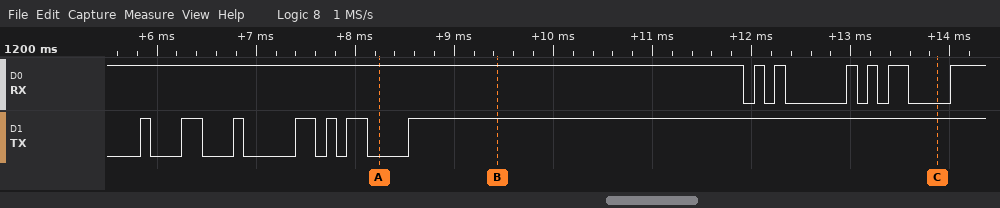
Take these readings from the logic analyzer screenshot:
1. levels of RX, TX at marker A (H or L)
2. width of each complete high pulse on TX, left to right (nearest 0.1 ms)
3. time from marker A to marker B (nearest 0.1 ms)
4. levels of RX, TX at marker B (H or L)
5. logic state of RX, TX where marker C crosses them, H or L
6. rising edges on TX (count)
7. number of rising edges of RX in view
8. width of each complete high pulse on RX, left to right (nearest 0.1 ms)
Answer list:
RX=H, TX=L
0.1 ms, 0.2 ms, 0.1 ms, 0.2 ms, 0.1 ms, 0.2 ms
1.2 ms
RX=H, TX=H
RX=L, TX=H
7
6
0.1 ms, 0.1 ms, 0.1 ms, 0.1 ms, 0.2 ms
